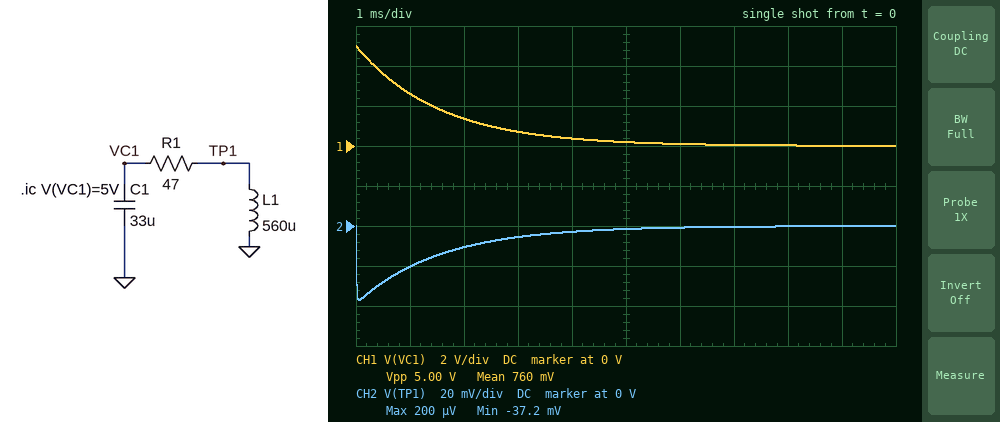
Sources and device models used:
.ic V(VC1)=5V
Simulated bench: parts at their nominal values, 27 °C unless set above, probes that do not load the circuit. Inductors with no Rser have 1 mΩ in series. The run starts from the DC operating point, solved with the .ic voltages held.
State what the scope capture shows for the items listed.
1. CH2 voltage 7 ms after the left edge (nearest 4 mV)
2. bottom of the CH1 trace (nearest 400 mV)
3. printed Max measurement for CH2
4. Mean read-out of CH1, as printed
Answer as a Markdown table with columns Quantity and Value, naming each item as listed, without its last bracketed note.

| Quantity | Value |
|---|---|
| CH2 voltage 7 ms after the left edge | 0 V |
| bottom of the CH1 trace | 0 V |
| printed Max measurement for CH2 | 200 µV |
| Mean read-out of CH1, as printed | 760 mV |
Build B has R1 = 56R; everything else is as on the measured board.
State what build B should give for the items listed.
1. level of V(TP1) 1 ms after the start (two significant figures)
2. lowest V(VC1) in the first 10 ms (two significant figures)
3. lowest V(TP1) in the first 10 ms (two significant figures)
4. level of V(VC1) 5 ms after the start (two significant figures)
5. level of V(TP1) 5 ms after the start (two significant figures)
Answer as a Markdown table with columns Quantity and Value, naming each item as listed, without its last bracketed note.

| Quantity | Value |
|---|---|
| level of V(TP1) 1 ms after the start | -16 mV |
| lowest V(VC1) in the first 10 ms | 22 mV |
| lowest V(TP1) in the first 10 ms | -26 mV |
| level of V(VC1) 5 ms after the start | 330 mV |
| level of V(TP1) 5 ms after the start | -1.8 mV |
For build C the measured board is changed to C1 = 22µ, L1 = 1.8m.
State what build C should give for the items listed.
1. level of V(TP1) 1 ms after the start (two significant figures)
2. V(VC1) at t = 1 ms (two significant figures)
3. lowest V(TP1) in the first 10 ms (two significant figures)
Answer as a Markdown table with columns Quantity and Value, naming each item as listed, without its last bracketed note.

| Quantity | Value |
|---|---|
| level of V(TP1) 1 ms after the start | -73 mV |
| V(VC1) at t = 1 ms | 1.8 V |
| lowest V(TP1) in the first 10 ms | -170 mV |
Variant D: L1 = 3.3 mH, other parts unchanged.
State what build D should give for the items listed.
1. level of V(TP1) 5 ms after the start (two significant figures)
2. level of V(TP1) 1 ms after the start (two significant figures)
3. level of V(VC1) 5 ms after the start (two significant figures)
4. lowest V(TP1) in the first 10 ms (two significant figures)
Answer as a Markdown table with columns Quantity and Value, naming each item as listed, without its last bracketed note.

| Quantity | Value |
|---|---|
| level of V(TP1) 5 ms after the start | -8.5 mV |
| level of V(TP1) 1 ms after the start | -130 mV |
| level of V(VC1) 5 ms after the start | 170 mV |
| lowest V(TP1) in the first 10 ms | -200 mV |
